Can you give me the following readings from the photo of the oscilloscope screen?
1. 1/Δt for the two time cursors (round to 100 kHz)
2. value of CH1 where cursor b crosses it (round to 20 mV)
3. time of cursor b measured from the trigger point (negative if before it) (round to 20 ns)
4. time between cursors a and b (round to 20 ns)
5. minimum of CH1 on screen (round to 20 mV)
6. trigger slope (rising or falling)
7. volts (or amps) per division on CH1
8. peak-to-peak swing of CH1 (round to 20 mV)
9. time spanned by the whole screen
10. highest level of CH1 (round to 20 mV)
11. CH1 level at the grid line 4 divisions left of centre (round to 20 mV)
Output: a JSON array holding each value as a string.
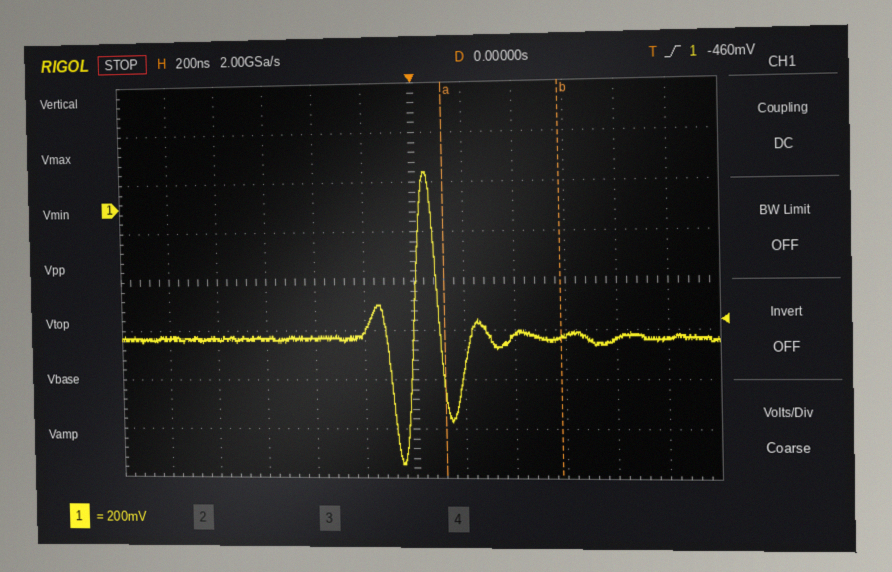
["2.2 MHz", "-520 mV", "+580 ns", "460 ns", "-1.04 V", "rising", "200 mV", "1.18 V", "2.4 µs", "140 mV", "-540 mV"]
